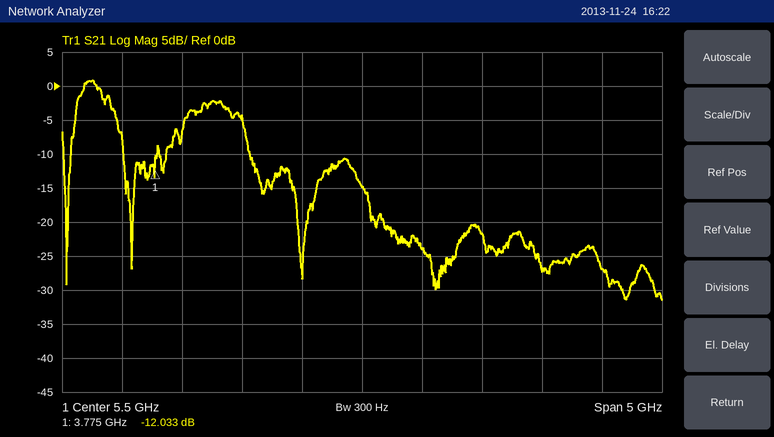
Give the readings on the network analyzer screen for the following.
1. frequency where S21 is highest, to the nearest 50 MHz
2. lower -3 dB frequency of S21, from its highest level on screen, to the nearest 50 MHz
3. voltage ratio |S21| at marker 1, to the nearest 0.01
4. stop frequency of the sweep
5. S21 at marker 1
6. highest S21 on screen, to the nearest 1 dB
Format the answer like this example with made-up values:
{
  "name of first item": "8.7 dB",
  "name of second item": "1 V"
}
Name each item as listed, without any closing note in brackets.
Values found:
{
  "frequency where S21 is highest, to the nearest 50 MHz": "3.25 GHz",
  "lower -3 dB frequency of S21, from its highest level on screen, to the nearest 50 MHz": "3.15 GHz",
  "voltage ratio |S21| at marker 1, to the nearest 0.01": "0.25",
  "stop frequency of the sweep": "8 GHz",
  "S21 at marker 1": "-12.033 dB",
  "highest S21 on screen, to the nearest 1 dB": "1 dB"
}
